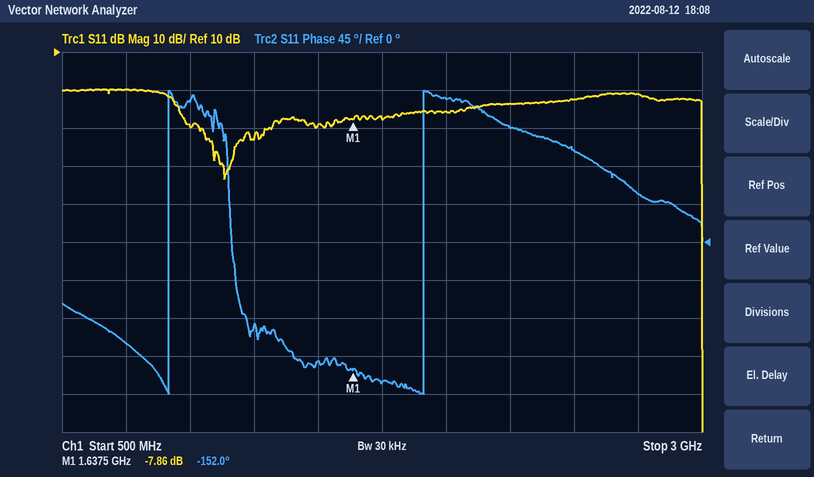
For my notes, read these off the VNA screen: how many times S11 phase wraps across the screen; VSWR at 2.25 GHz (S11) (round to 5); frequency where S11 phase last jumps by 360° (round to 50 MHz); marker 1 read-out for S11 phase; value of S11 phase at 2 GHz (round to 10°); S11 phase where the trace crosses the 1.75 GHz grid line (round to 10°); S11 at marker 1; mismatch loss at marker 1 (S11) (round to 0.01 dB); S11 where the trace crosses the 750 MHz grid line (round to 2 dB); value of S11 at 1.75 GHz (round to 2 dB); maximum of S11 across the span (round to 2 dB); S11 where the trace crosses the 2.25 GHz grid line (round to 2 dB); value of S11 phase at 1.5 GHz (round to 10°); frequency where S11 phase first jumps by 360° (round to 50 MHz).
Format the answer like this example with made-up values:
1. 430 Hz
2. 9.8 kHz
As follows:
1. 2
2. 5
3. 1.90 GHz
4. -152.0°
5. 170°
6. -170°
7. -7.86 dB
8. 0.78 dB
9. 0 dB
10. -8 dB
11. 0 dB
12. -4 dB
13. -140°
14. 900 MHz
